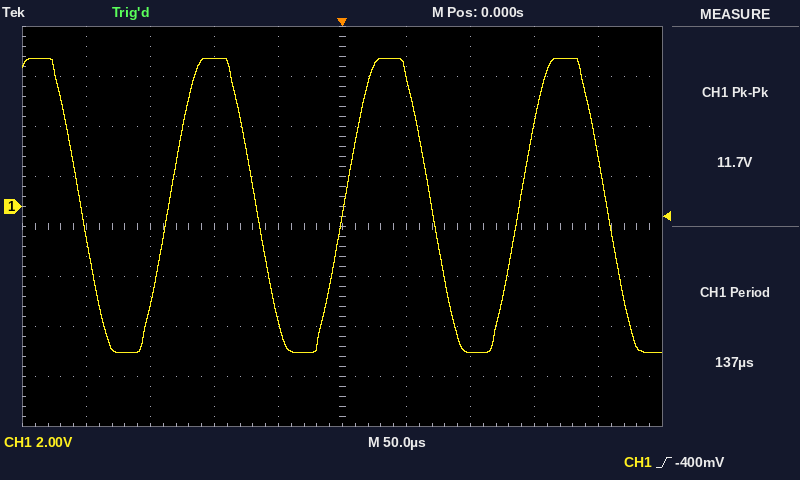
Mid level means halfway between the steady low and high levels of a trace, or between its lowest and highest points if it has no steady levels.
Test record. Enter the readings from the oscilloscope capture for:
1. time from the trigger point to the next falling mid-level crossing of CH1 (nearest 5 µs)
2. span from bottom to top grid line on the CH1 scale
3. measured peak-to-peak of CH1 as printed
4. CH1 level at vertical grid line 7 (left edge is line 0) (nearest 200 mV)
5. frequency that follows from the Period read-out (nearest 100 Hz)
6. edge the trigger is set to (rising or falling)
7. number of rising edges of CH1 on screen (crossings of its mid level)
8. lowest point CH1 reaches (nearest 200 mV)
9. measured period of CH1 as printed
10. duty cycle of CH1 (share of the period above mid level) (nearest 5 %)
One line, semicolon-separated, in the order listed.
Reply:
70 µs; 16 V; 11.7 V; -5.8 V; 7.3 kHz; rising; 3; -5.8 V; 137 µs; 50 %
